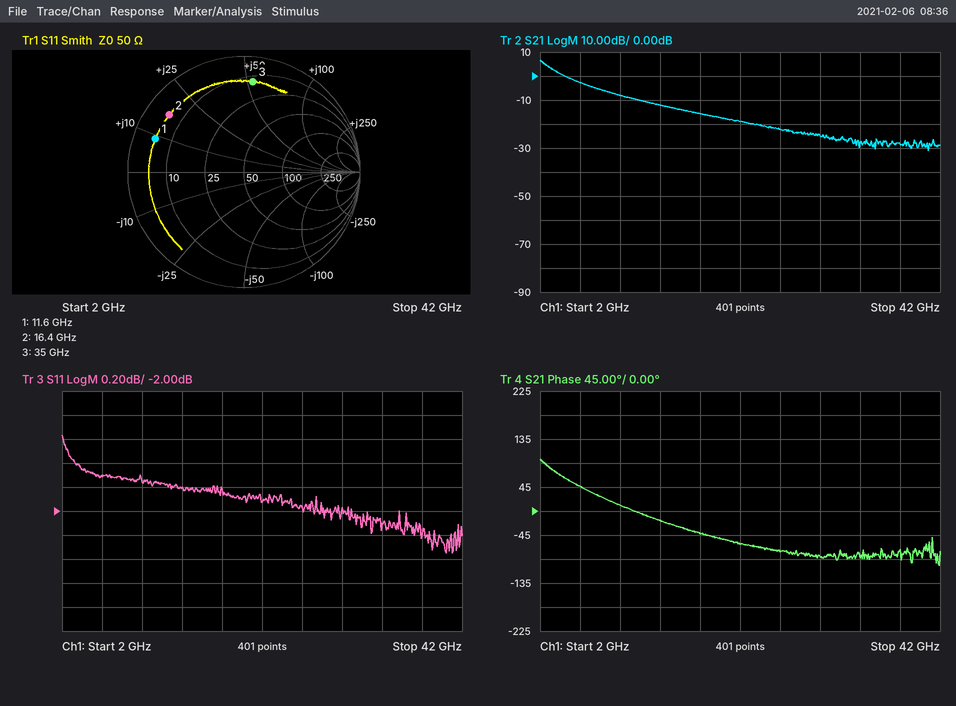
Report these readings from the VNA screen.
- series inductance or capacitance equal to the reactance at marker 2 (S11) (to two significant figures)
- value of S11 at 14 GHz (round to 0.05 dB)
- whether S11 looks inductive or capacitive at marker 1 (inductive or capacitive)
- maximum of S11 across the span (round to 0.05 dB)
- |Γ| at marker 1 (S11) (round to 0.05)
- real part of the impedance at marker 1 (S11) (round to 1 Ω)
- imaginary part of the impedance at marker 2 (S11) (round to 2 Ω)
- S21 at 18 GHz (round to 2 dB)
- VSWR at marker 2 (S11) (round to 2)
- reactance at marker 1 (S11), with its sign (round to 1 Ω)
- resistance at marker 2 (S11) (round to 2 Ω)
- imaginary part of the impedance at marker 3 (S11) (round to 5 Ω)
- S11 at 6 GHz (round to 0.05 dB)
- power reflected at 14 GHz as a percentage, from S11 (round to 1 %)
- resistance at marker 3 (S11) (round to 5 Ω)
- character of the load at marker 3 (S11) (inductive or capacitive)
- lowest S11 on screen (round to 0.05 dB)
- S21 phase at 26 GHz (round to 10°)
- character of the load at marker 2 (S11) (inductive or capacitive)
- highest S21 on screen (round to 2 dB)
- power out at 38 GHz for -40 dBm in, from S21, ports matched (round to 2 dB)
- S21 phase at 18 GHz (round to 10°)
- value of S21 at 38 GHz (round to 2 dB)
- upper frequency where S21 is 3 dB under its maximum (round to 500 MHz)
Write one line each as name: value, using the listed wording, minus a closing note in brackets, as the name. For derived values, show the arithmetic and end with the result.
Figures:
series inductance or capacitance equal to the reactance at marker 2 (S11): L = 16 Ω/(2π × 16.4 GHz) ≈ 155 pH, so 160 pH to two significant figures
value of S11 at 14 GHz: -1.80 dB
whether S11 looks inductive or capacitive at marker 1: inductive
maximum of S11 across the span: -1.35 dB
|Γ| at marker 1 (S11): 0.80
real part of the impedance at marker 1 (S11): 5 Ω
imaginary part of the impedance at marker 2 (S11): +16 Ω
S21 at 18 GHz: -16 dB
VSWR at marker 2 (S11): 10
reactance at marker 1 (S11), with its sign: +9 Ω
resistance at marker 2 (S11): 6 Ω
imaginary part of the impedance at marker 3 (S11): +55 Ω
S11 at 6 GHz: -1.70 dB
power reflected at 14 GHz as a percentage, from S11: 10^(-1.8/10) ≈ 66 %
resistance at marker 3 (S11): 15 Ω
character of the load at marker 3 (S11): inductive
lowest S11 on screen: -2.35 dB
S21 phase at 26 GHz: -80°
character of the load at marker 2 (S11): inductive
highest S21 on screen: 6 dB
power out at 38 GHz for -40 dBm in, from S21, ports matched: -40 dBm + (-28 dB) = -68 dBm
S21 phase at 18 GHz: -40°
value of S21 at 38 GHz: -28 dB
upper frequency where S21 is 3 dB under its maximum: 3.0 GHz
